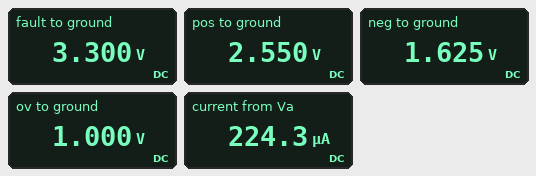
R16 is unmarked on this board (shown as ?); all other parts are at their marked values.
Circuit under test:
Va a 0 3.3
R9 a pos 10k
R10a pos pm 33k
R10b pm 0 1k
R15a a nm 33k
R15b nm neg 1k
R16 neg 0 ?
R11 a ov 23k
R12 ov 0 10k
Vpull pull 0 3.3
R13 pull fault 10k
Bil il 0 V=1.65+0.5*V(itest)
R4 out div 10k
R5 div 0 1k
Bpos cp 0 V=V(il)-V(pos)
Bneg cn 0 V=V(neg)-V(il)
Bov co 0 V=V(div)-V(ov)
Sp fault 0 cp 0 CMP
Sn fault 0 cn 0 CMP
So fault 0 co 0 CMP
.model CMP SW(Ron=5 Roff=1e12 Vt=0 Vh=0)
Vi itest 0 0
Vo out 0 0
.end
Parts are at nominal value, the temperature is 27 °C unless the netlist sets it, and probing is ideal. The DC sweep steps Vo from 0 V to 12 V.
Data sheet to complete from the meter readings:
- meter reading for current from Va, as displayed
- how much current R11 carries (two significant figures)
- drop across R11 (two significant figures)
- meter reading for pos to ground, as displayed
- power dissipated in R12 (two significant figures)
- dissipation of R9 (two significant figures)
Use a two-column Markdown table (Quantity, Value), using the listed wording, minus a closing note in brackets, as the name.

| Quantity | Value |
|---|---|
| meter reading for current from Va, as displayed | 224.3 µA |
| how much current R11 carries | 100 µA |
| drop across R11 | 2.3 V |
| meter reading for pos to ground, as displayed | 2.550 V |
| power dissipated in R12 | 100 µW |
| dissipation of R9 | 56 µW |
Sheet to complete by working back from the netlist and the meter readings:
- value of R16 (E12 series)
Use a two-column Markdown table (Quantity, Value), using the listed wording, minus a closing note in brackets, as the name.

| Quantity | Value |
|---|---|
| value of R16 | 33 kΩ |
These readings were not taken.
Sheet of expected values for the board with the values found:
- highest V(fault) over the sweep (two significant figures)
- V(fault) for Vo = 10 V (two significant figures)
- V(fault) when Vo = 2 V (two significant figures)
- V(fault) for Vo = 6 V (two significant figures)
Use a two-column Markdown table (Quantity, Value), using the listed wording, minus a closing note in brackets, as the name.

| Quantity | Value |
|---|---|
| highest V(fault) over the sweep | 3.3 V |
| V(fault) for Vo = 10 V | 3.3 V |
| V(fault) when Vo = 2 V | 3.3 V |
| V(fault) for Vo = 6 V | 3.3 V |
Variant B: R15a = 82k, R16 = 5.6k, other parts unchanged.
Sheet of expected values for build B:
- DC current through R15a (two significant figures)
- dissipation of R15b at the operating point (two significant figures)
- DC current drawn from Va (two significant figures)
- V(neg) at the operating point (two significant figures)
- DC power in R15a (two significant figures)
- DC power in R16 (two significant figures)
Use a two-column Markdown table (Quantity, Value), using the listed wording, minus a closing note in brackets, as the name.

| Quantity | Value |
|---|---|
| DC current through R15a | 37 µA |
| dissipation of R15b at the operating point | 1.4 µW |
| DC current drawn from Va | 210 µA |
| V(neg) at the operating point | 210 mV |
| DC power in R15a | 110 µW |
| DC power in R16 | 7.8 µW |
